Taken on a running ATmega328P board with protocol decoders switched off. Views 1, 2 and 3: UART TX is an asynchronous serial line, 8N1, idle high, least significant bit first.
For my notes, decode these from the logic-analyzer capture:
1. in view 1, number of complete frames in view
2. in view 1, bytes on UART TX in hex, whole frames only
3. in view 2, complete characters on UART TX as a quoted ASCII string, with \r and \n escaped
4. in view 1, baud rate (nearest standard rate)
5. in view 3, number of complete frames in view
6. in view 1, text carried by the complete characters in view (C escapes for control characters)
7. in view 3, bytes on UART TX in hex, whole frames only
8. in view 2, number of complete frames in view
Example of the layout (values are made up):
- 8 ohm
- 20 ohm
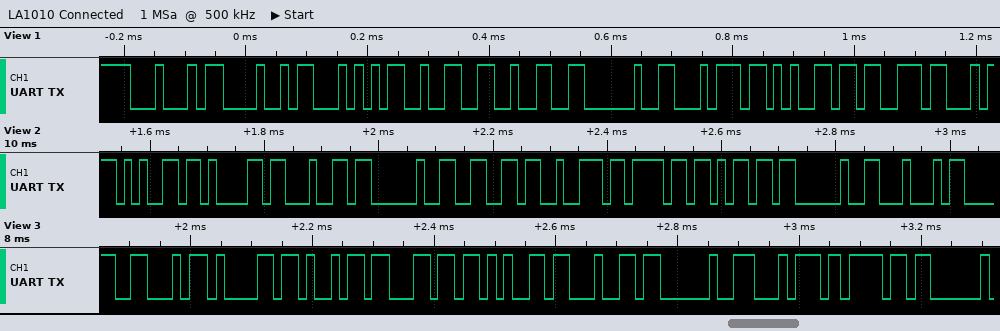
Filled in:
- 9
- 44 48 54 32 32 20 74 65 73
- "ead from D"
- 74880 baud
- 9
- "DHT22 tes"
- 46 61 69 6C 65 64 20 74 6F
- 10
